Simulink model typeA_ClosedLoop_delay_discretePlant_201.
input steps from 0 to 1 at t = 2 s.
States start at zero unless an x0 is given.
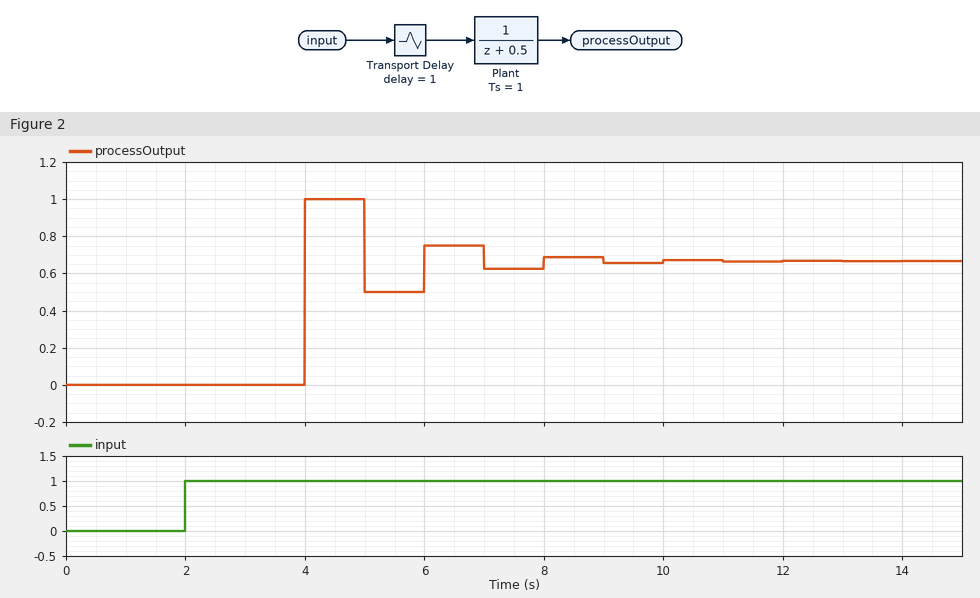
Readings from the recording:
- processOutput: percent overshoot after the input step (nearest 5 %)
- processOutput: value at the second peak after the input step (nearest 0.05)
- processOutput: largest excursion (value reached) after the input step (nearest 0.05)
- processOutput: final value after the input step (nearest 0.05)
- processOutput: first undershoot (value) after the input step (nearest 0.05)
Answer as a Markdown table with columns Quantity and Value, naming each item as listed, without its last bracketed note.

| Quantity | Value |
|---|---|
| processOutput: percent overshoot after the input step | 50 % |
| processOutput: value at the second peak after the input step | 0.75 |
| processOutput: largest excursion (value reached) after the input step | 1.00 |
| processOutput: final value after the input step | 0.65 |
| processOutput: first undershoot (value) after the input step | 0.50 |
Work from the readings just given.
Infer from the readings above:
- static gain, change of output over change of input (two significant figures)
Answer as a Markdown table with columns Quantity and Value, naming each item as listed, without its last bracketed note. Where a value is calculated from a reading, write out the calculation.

| Quantity | Value |
|---|---|
| static gain, change of output over change of input | (0.65 - 0) / (1 - 0) = 0.65 |
